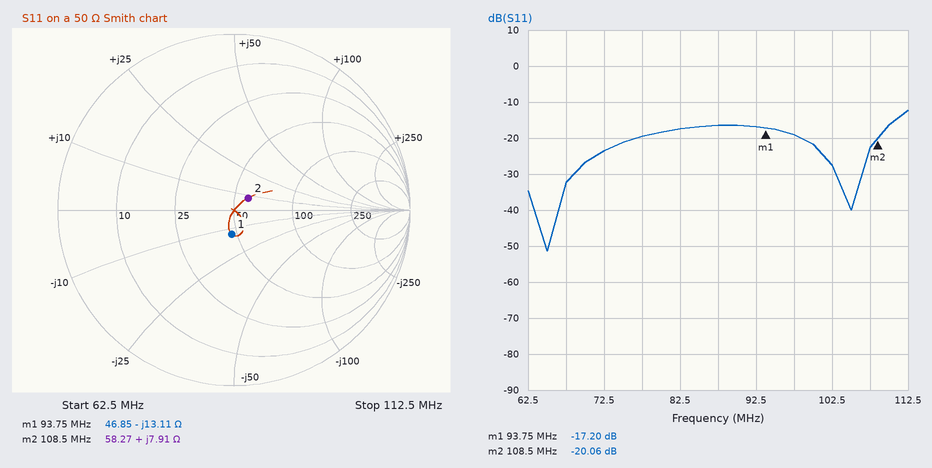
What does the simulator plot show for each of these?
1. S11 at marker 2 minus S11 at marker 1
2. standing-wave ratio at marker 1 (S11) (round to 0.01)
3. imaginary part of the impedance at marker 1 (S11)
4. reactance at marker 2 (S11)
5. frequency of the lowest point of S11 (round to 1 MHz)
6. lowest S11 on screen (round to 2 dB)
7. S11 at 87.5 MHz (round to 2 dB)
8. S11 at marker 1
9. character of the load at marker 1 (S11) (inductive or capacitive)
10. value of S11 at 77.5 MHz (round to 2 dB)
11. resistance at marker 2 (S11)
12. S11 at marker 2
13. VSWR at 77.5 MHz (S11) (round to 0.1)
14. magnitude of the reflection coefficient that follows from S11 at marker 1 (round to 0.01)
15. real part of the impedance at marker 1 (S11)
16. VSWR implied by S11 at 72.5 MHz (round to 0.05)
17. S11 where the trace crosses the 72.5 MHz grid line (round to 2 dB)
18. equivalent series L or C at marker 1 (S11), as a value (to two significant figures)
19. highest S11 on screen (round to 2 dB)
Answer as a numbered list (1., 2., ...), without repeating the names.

1. -2.86 dB
2. 1.32
3. -13.11 Ω
4. +7.91 Ω
5. 65 MHz
6. -52 dB
7. -16 dB
8. -17.20 dB
9. capacitive
10. -20 dB
11. 58.27 Ω
12. -20.06 dB
13. 1.2
14. 0.14
15. 46.85 Ω
16. 1.15
17. -24 dB
18. 130 pF
19. -12 dB
